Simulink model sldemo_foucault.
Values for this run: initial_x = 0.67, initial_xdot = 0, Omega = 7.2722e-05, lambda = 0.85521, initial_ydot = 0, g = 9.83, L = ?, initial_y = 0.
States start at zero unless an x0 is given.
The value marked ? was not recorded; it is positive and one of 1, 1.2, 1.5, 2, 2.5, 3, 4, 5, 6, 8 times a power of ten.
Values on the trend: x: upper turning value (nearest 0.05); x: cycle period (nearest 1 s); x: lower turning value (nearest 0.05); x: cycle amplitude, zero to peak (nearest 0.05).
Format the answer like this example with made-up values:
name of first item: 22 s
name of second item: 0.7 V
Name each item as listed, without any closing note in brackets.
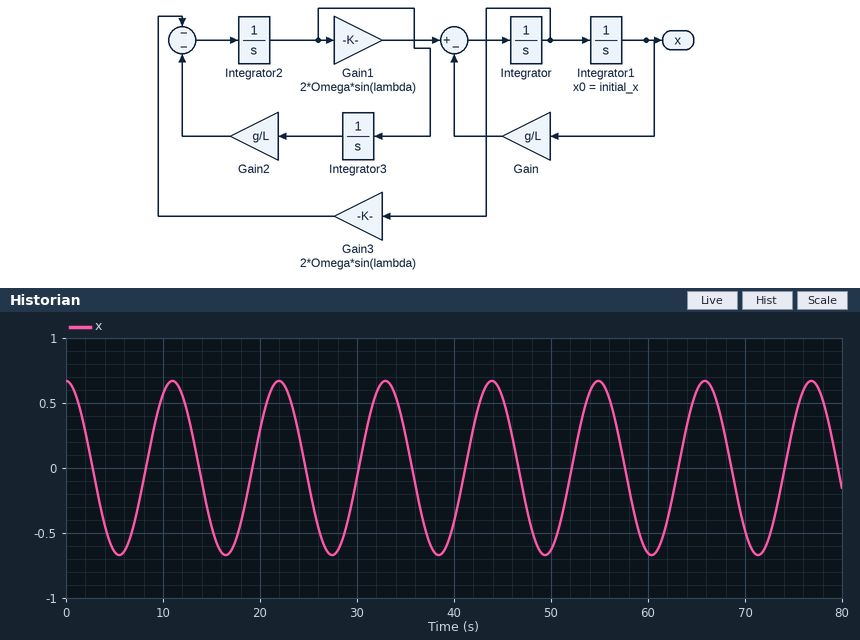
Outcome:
x: upper turning value: 0.65
x: cycle period: 11 s
x: lower turning value: -0.65
x: cycle amplitude, zero to peak: 0.65
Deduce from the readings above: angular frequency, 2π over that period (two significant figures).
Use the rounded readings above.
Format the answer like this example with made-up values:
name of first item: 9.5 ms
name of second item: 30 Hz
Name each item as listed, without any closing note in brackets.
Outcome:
angular frequency, 2π over that period: 0.57 rad/s
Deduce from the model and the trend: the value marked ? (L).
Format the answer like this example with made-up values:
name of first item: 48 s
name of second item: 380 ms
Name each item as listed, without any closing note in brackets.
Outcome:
the value marked ?: 30
